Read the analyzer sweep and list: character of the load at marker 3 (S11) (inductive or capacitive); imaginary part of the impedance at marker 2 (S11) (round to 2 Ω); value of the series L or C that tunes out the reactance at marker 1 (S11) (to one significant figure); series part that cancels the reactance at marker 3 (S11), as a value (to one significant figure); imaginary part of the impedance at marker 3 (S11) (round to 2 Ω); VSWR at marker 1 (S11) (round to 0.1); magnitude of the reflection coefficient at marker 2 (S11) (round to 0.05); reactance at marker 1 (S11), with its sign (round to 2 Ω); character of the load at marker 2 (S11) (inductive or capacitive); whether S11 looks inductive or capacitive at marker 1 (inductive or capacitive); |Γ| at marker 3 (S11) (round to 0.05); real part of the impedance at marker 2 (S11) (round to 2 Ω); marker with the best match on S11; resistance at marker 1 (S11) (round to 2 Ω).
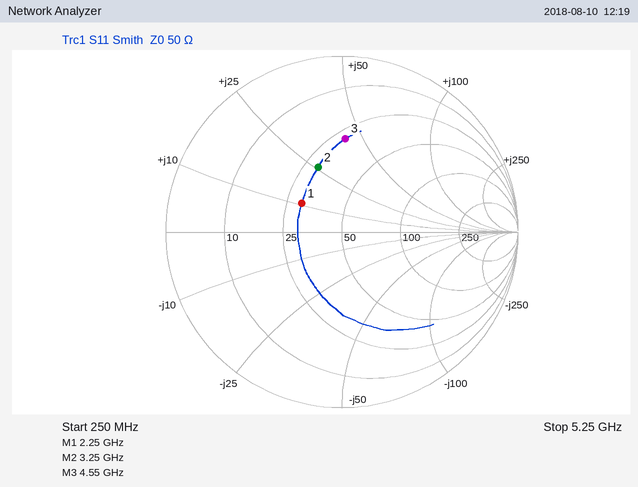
inductive
+26 Ω
7 pF
800 fF
+42 Ω
1.8
0.40
+10 Ω
inductive
inductive
0.55
30 Ω
marker 1
30 Ω
